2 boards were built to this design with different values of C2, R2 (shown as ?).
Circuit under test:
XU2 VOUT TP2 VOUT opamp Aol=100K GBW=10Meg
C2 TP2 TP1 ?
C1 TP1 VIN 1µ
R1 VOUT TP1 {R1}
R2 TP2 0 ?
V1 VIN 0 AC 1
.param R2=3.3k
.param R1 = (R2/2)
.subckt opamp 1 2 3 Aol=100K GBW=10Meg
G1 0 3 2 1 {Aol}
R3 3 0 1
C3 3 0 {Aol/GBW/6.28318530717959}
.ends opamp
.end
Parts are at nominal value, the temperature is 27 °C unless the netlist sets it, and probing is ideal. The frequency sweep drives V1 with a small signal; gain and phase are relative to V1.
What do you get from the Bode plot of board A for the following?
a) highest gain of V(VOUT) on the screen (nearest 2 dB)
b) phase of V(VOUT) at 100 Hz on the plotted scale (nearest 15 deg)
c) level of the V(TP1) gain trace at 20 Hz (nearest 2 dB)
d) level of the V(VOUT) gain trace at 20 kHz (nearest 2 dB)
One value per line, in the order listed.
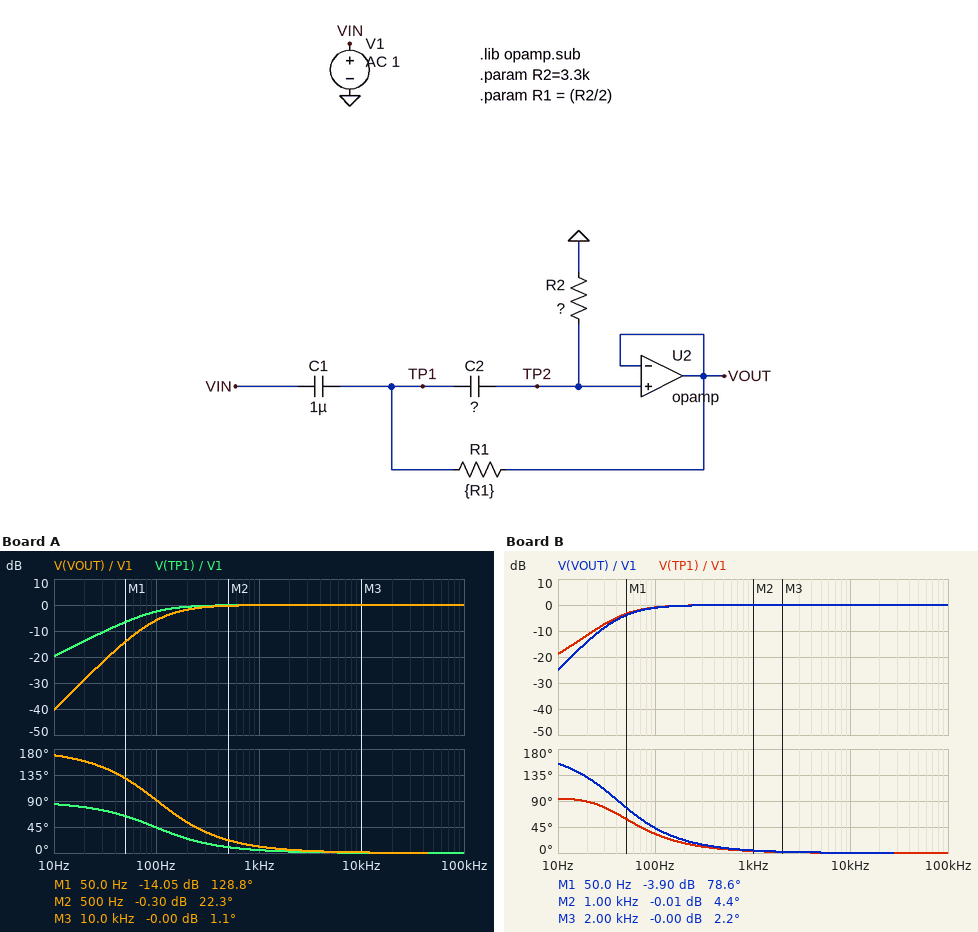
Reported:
0 dB
90 deg
-14 dB
0 dB
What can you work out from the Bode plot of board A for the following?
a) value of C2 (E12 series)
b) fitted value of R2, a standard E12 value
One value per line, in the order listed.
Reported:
820 nF
1.8 kΩ
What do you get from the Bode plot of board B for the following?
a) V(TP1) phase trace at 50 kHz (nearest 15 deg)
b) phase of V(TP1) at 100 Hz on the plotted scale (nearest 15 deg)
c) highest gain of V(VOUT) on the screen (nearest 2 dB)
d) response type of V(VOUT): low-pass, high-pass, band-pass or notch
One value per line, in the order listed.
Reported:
0 deg
30 deg
0 dB
high-pass
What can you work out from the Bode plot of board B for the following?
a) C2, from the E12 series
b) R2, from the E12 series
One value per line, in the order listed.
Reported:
3.3 µF
2.7 kΩ
